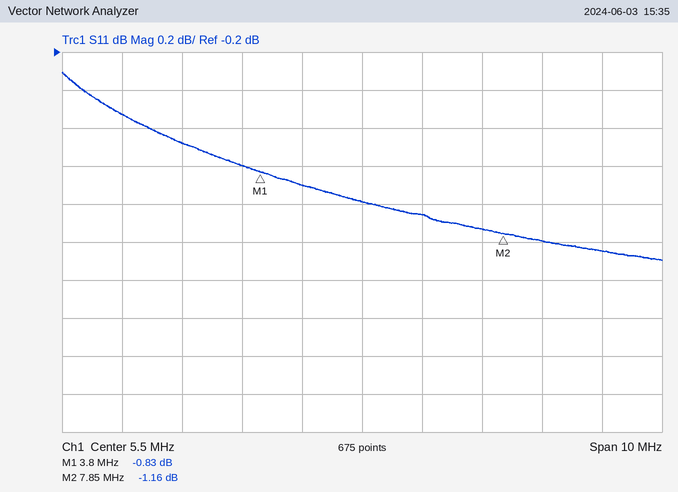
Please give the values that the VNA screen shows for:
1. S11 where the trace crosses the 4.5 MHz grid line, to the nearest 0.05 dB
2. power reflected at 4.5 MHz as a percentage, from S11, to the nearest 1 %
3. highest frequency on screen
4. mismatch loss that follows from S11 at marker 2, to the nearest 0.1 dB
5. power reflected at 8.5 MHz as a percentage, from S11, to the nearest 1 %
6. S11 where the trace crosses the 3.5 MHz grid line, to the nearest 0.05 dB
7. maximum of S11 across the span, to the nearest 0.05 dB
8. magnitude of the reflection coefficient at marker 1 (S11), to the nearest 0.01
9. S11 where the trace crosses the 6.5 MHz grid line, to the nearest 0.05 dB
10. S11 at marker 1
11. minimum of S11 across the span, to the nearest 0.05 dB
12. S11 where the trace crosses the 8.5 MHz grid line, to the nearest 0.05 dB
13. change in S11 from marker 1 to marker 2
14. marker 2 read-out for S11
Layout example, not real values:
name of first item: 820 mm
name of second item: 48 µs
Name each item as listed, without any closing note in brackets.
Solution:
S11 where the trace crosses the 4.5 MHz grid line, to the nearest 0.05 dB: -0.90 dB
power reflected at 4.5 MHz as a percentage, from S11, to the nearest 1 %: 81 %
highest frequency on screen: 10.5 MHz
mismatch loss that follows from S11 at marker 2, to the nearest 0.1 dB: 6.3 dB
power reflected at 8.5 MHz as a percentage, from S11, to the nearest 1 %: 76 %
S11 where the trace crosses the 3.5 MHz grid line, to the nearest 0.05 dB: -0.80 dB
maximum of S11 across the span, to the nearest 0.05 dB: -0.30 dB
magnitude of the reflection coefficient at marker 1 (S11), to the nearest 0.01: 0.91
S11 where the trace crosses the 6.5 MHz grid line, to the nearest 0.05 dB: -1.05 dB
S11 at marker 1: -0.83 dB
minimum of S11 across the span, to the nearest 0.05 dB: -1.30 dB
S11 where the trace crosses the 8.5 MHz grid line, to the nearest 0.05 dB: -1.20 dB
change in S11 from marker 1 to marker 2: -0.33 dB
marker 2 read-out for S11: -1.16 dB
